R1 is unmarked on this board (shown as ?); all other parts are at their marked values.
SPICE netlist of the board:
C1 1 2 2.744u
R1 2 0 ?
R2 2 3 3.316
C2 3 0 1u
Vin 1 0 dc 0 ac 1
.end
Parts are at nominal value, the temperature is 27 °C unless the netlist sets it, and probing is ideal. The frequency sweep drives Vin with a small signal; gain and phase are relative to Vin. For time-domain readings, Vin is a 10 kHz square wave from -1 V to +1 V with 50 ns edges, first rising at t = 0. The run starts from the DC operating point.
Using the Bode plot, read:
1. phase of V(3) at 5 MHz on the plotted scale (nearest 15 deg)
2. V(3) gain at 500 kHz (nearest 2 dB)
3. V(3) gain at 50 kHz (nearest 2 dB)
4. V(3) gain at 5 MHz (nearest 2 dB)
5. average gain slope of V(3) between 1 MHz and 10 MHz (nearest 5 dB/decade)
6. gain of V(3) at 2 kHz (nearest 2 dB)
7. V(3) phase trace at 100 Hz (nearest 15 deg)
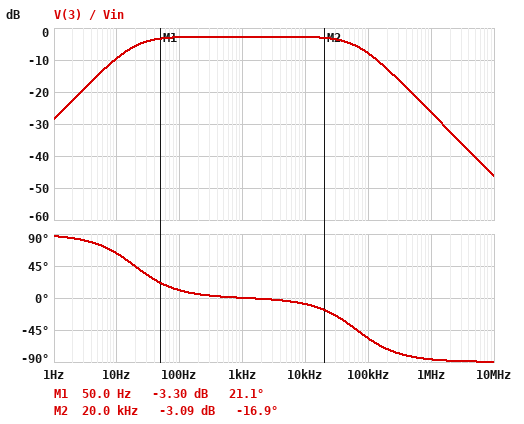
-90 deg
-20 dB
-4 dB
-40 dB
-20 dB/decade
-2 dB
15 deg
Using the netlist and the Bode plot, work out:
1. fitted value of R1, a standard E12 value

2.2 kΩ
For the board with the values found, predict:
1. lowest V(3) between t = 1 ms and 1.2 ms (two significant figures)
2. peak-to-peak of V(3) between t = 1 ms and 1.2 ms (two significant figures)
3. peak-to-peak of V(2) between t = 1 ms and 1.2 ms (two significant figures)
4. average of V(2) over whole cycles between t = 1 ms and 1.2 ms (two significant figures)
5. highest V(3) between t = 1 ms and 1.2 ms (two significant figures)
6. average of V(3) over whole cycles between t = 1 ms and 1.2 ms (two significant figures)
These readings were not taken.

-99 mV
1.5 V
2.5 V
640 mV
1.4 V
640 mV
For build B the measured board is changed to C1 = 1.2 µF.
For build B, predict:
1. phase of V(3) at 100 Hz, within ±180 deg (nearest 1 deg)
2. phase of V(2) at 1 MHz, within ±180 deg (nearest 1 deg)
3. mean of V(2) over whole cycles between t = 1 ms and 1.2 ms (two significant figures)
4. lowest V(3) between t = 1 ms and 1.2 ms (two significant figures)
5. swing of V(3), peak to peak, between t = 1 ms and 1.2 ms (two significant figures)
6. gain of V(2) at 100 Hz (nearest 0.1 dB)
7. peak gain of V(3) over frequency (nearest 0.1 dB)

18 deg
2 deg
430 mV
-120 mV
1.1 V
-5.7 dB
-5.3 dB
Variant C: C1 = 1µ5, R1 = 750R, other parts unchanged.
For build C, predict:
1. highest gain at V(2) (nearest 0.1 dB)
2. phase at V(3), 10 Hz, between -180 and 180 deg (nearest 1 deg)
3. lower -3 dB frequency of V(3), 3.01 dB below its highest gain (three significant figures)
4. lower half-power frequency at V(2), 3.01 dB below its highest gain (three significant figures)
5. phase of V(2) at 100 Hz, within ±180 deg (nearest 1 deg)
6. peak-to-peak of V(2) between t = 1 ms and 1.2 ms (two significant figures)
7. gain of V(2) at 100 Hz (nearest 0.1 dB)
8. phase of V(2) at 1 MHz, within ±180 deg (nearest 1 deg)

0 dB
83 deg
84.6 Hz
42.4 kHz
40 deg
2.8 V
-6.8 dB
2 deg
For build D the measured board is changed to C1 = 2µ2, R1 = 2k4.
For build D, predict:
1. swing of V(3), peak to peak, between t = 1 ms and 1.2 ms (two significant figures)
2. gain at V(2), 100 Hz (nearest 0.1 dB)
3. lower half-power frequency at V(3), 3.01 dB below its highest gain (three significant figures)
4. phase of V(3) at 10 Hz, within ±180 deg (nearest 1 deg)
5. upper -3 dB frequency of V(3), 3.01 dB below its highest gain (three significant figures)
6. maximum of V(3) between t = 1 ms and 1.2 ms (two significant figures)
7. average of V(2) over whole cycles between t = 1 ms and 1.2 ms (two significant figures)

1.4 V
-3.4 dB
20.7 Hz
64 deg
69.9 kHz
1.3 V
590 mV
